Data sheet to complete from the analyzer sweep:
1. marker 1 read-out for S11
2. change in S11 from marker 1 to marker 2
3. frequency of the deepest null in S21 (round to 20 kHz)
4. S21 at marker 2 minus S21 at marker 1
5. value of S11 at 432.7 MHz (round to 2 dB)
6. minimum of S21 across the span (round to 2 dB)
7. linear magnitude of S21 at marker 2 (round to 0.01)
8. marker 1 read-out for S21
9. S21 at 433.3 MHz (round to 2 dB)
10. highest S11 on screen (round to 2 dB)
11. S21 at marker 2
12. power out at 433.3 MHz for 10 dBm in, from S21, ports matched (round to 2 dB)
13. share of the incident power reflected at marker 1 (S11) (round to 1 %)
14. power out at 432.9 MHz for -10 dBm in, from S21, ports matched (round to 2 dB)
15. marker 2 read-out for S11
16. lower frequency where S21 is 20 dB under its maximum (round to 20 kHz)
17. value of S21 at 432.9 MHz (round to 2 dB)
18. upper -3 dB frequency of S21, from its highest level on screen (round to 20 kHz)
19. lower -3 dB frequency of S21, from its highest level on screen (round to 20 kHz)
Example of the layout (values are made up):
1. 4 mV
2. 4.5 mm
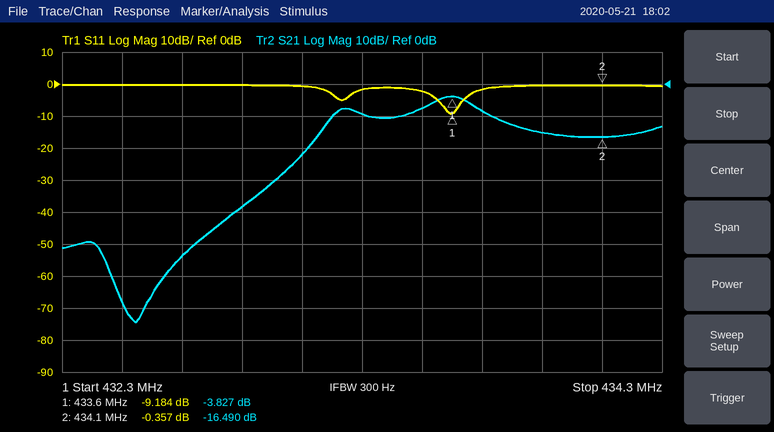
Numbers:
1. -9.184 dB
2. 8.827 dB
3. 432.54 MHz
4. -12.663 dB
5. 0 dB
6. -74 dB
7. 0.15
8. -3.827 dB
9. -10 dB
10. 0 dB
11. -16.490 dB
12. 0 dBm
13. 12 %
14. -48 dBm
15. -0.357 dB
16. 433.08 MHz
17. -38 dB
18. 433.68 MHz
19. 433.52 MHz
